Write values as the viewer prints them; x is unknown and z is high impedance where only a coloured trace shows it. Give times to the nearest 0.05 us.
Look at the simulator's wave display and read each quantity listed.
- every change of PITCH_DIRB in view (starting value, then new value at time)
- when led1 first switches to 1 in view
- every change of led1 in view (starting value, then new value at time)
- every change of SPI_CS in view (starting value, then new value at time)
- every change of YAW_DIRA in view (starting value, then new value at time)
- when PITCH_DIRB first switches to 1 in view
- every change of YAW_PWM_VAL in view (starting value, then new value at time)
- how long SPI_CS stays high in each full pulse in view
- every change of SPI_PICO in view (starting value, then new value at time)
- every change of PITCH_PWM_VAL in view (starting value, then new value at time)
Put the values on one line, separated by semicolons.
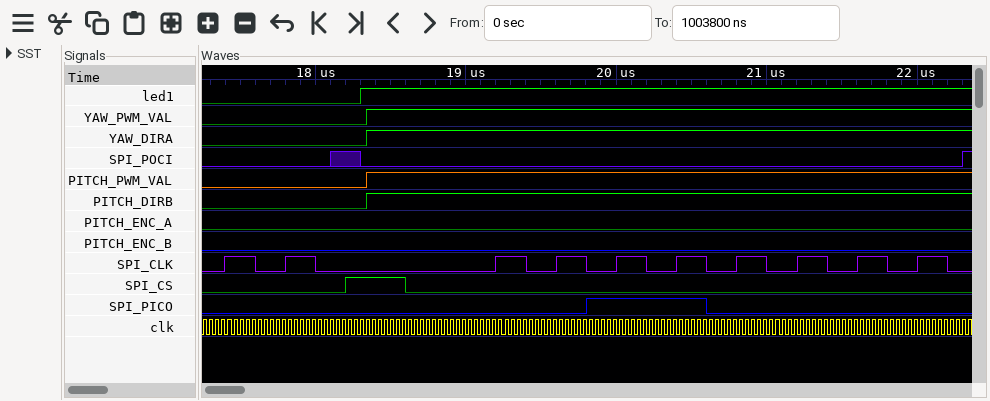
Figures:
0, 1 at 18.35 us; 18.3 us; 0, 1 at 18.3 us; 0, 1 at 18.2 us, 0 at 18.6 us; 0, 1 at 18.35 us; 18.35 us; 0, 1 at 18.35 us; 0.4 us; 0, 1 at 19.8 us, 0 at 20.6 us; 0, 1 at 18.35 us
